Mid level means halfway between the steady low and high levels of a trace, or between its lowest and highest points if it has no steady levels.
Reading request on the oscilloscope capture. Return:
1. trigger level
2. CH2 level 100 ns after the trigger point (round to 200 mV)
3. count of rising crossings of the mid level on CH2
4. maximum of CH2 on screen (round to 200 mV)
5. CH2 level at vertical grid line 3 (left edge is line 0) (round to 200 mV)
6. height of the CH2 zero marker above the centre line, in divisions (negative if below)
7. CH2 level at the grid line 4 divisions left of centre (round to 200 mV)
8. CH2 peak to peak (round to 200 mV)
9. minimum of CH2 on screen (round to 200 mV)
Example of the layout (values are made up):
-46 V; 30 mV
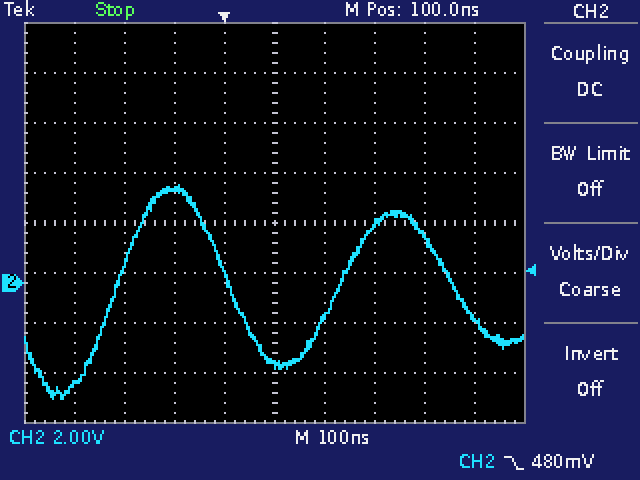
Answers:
480 mV; -3.2 V; 2; 4.0 V; 3.8 V; -1.2 div; -4.0 V; 8.6 V; -4.6 V
